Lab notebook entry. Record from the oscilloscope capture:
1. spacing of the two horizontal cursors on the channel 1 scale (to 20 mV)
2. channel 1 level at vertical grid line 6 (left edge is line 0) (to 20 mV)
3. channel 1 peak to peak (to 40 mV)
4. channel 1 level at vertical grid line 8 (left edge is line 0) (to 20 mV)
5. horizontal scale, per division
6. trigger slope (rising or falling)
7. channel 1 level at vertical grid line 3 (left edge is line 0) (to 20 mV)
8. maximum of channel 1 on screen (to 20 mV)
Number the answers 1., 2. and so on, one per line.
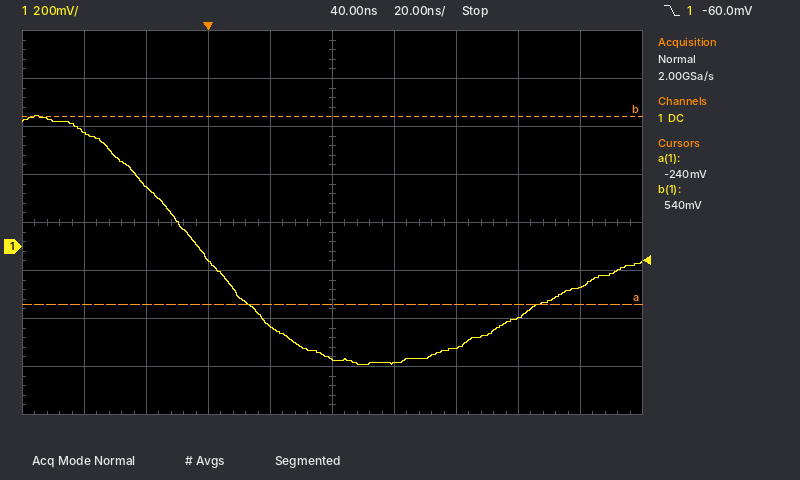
1. 780 mV
2. -480 mV
3. 1.04 V
4. -300 mV
5. 20 ns
6. falling
7. -60 mV
8. 540 mV
